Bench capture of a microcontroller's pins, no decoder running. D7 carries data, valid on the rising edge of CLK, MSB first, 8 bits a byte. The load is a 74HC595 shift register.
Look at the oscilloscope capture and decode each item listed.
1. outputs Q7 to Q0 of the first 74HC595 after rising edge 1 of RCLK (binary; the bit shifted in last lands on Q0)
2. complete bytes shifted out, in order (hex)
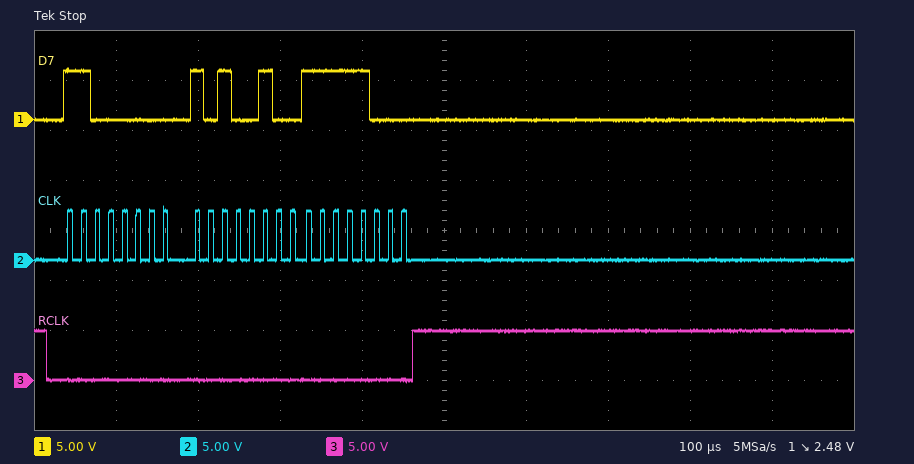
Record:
11111000
C0 A4 F8
